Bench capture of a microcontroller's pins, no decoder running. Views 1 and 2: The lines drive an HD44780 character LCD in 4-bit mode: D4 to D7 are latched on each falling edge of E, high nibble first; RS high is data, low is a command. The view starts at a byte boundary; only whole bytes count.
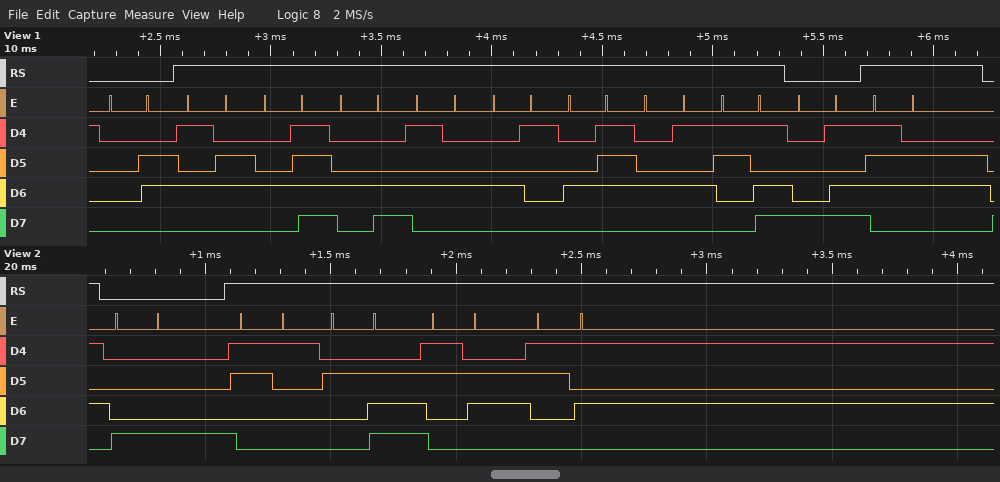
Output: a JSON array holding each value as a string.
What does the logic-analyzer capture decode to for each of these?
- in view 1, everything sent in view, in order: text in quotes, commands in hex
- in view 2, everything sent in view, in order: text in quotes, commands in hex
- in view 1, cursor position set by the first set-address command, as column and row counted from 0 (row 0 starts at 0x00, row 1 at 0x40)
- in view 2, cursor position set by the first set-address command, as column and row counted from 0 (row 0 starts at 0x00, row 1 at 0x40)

["0x06 \"VOLTAGE=\" 0x8D \"v\"", "0x88 \"1.65\"", "column 13, row 0", "column 8, row 0"]
